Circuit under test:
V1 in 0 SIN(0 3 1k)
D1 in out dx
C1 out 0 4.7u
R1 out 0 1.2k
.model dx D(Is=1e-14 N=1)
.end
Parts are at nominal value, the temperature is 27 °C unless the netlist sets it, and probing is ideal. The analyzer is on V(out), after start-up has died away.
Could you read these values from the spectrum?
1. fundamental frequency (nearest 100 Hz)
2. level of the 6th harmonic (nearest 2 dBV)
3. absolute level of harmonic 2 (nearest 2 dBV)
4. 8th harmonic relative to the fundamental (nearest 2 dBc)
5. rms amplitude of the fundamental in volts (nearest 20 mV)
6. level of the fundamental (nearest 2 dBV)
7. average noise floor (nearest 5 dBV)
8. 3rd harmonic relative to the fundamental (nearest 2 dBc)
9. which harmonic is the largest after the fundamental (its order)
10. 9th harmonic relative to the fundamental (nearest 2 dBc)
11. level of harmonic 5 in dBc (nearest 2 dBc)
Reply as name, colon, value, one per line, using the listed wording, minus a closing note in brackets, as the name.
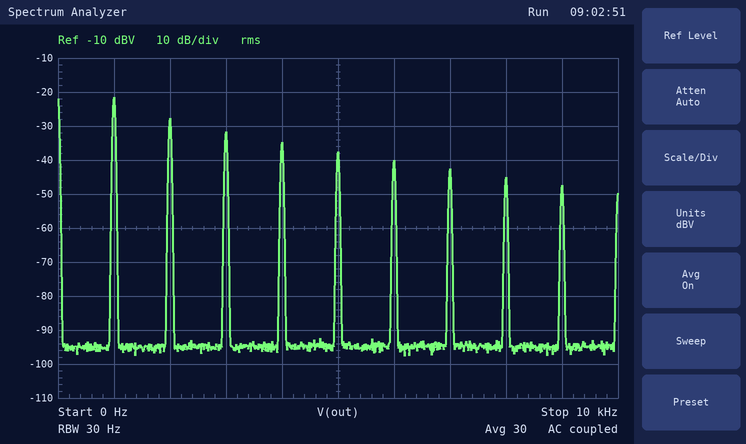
fundamental frequency: 1.0 kHz
level of the 6th harmonic: -40 dBV
absolute level of harmonic 2: -28 dBV
8th harmonic relative to the fundamental: -24 dBc
rms amplitude of the fundamental in volts: 80 mV
level of the fundamental: -22 dBV
average noise floor: -95 dBV
3rd harmonic relative to the fundamental: -10 dBc
which harmonic is the largest after the fundamental: 2
9th harmonic relative to the fundamental: -26 dBc
level of harmonic 5 in dBc: -16 dBc
